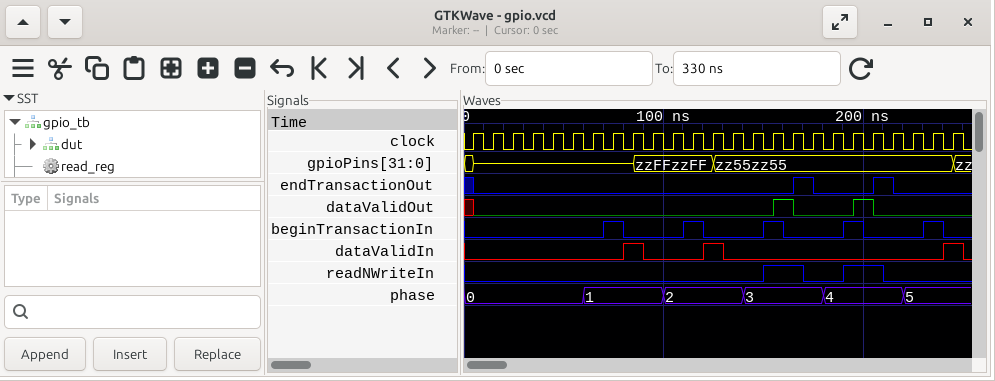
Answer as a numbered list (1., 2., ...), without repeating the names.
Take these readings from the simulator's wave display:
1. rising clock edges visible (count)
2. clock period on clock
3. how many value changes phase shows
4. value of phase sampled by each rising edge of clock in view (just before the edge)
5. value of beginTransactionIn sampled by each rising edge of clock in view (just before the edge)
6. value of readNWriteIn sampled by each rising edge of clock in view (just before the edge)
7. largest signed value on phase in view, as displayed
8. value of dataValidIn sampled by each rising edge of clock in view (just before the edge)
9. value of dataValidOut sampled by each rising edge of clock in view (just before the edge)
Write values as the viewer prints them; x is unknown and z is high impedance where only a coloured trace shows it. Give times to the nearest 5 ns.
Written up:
1. 25
2. 10 ns
3. 5
4. 0, 0, 0, 0, 0, 0, 1, 1, 1, 1, 2, 2, 2, 2, 3, 3, 3, 3, 4, 4, 4, 4, 5, 5, 5
5. 0 0 0 0 0 0 0 1 0 0 0 1 0 0 0 1 0 0 0 1 0 0 0 1 0
6. 0 0 0 0 0 0 0 0 0 0 0 0 0 0 0 1 1 0 0 1 1 0 0 0 0
7. 5
8. 0 0 0 0 0 0 0 0 1 0 0 0 1 0 0 0 0 0 0 0 0 0 0 0 1
9. x 0 0 0 0 0 0 0 0 0 0 0 0 0 0 0 1 0 0 0 1 0 0 0 0
